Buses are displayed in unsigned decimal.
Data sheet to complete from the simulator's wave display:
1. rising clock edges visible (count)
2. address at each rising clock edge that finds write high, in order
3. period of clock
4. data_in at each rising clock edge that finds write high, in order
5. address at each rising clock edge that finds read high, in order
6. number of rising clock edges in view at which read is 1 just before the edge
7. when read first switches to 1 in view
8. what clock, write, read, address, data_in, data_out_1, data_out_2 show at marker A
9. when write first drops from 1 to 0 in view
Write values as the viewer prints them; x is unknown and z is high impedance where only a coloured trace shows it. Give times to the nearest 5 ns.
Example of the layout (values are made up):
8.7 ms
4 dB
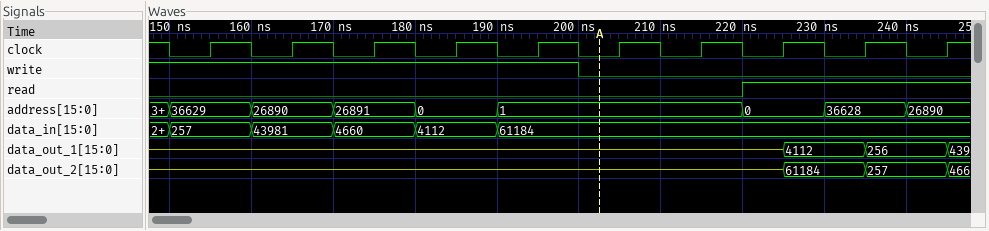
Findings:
10
36629, 26890, 26891, 0, 1
10 ns
257, 43981, 4660, 4112, 61184
0, 36628, 26890
3
220 ns
clock=0, write=0, read=0, address=1, data_in=61184, data_out_1=z, data_out_2=z
200 ns
